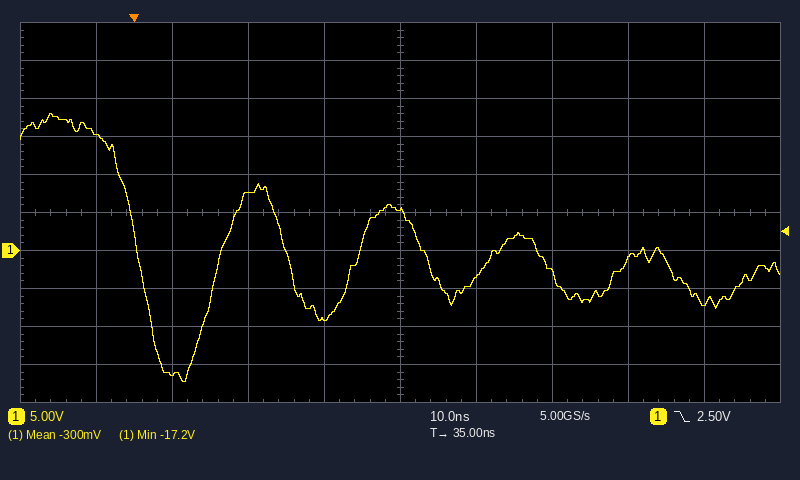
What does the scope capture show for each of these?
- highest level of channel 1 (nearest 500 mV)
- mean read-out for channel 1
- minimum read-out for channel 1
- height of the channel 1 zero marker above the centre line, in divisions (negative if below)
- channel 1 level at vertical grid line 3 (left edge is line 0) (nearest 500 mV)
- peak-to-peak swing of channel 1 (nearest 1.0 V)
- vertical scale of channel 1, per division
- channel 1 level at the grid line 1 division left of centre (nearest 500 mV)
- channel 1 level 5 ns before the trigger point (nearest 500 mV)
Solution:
18.0 V
-300 mV
-17.2 V
-1.0 div
7.5 V
35.0 V
5 V
-9.0 V
15.5 V
